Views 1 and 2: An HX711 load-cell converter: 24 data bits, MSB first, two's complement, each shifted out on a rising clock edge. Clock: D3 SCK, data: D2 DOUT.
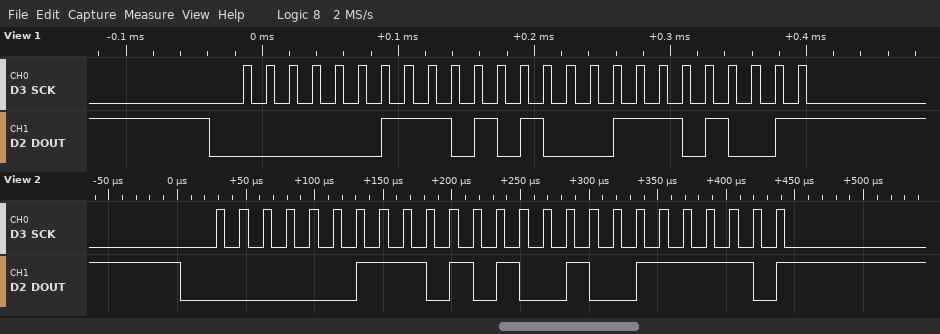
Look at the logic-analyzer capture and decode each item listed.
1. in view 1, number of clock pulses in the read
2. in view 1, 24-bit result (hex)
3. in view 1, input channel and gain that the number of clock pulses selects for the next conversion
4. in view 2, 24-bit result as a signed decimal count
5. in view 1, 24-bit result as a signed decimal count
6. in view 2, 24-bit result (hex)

25
0x03A8E9
channel A, gain 128
239934
239849
0x03A93E
